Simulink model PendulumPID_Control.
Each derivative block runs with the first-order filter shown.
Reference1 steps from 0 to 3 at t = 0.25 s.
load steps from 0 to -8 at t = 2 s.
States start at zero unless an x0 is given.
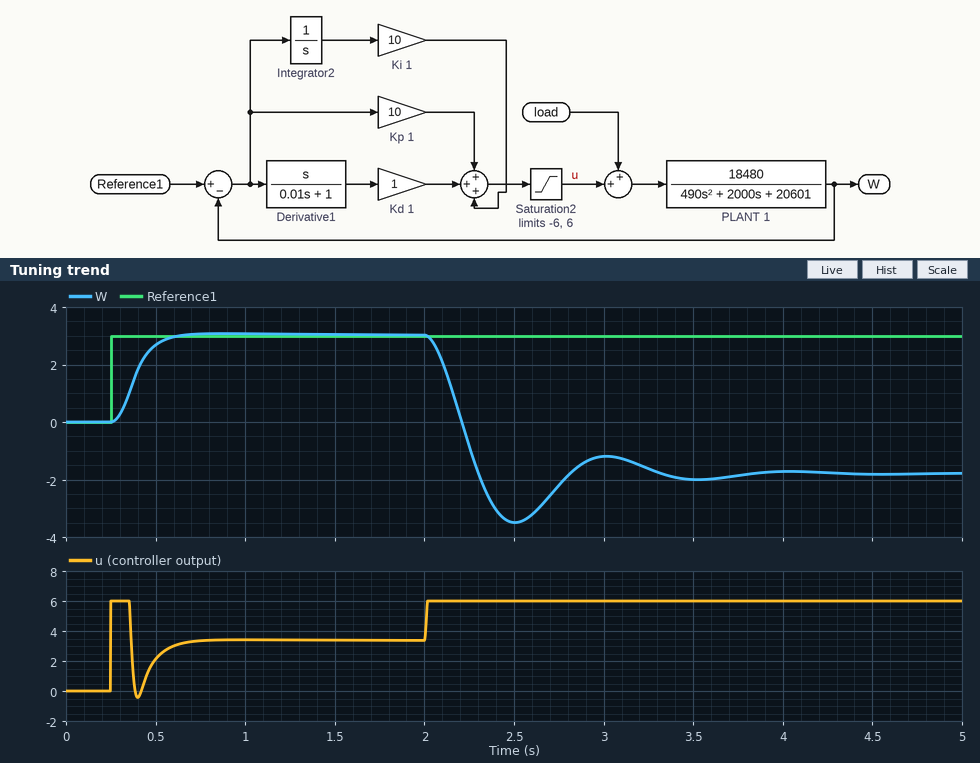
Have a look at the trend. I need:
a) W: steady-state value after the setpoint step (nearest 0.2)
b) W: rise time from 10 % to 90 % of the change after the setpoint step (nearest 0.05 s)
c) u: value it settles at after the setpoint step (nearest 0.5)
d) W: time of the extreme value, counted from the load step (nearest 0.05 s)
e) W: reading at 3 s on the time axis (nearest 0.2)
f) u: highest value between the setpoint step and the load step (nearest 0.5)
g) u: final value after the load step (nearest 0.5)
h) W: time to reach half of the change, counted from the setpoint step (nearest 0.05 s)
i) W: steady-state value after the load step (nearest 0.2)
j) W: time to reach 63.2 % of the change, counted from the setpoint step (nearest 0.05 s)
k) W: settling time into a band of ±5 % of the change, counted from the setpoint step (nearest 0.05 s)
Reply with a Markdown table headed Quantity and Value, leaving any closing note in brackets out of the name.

| Quantity | Value |
|---|---|
| W: steady-state value after the setpoint step | 3.0 |
| W: rise time from 10 % to 90 % of the change after the setpoint step | 0.20 s |
| u: value it settles at after the setpoint step | 3.5 |
| W: time of the extreme value, counted from the load step | 0.50 s |
| W: reading at 3 s on the time axis | -1.2 |
| u: highest value between the setpoint step and the load step | 6.0 |
| u: final value after the load step | 6.0 |
| W: time to reach half of the change, counted from the setpoint step | 0.15 s |
| W: steady-state value after the load step | -1.8 |
| W: time to reach 63.2 % of the change, counted from the setpoint step | 0.15 s |
| W: settling time into a band of ±5 % of the change, counted from the setpoint step | 0.30 s |
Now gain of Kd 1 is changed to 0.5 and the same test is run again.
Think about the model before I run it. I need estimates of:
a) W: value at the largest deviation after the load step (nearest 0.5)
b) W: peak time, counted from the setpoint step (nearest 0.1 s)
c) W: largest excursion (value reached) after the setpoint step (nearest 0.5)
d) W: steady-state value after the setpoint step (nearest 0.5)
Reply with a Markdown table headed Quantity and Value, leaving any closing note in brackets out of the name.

| Quantity | Value |
|---|---|
| W: value at the largest deviation after the load step | -3.5 |
| W: peak time, counted from the setpoint step | 0.3 s |
| W: largest excursion (value reached) after the setpoint step | 3.0 |
| W: steady-state value after the setpoint step | 3.0 |
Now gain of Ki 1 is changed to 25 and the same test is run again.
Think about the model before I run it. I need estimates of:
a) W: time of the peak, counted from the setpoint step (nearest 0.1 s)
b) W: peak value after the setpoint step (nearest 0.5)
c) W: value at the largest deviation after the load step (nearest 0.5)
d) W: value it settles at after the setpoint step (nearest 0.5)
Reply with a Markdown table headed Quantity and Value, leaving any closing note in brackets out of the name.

| Quantity | Value |
|---|---|
| W: time of the peak, counted from the setpoint step | 0.4 s |
| W: peak value after the setpoint step | 3.5 |
| W: value at the largest deviation after the load step | -3.5 |
| W: value it settles at after the setpoint step | 3.0 |
